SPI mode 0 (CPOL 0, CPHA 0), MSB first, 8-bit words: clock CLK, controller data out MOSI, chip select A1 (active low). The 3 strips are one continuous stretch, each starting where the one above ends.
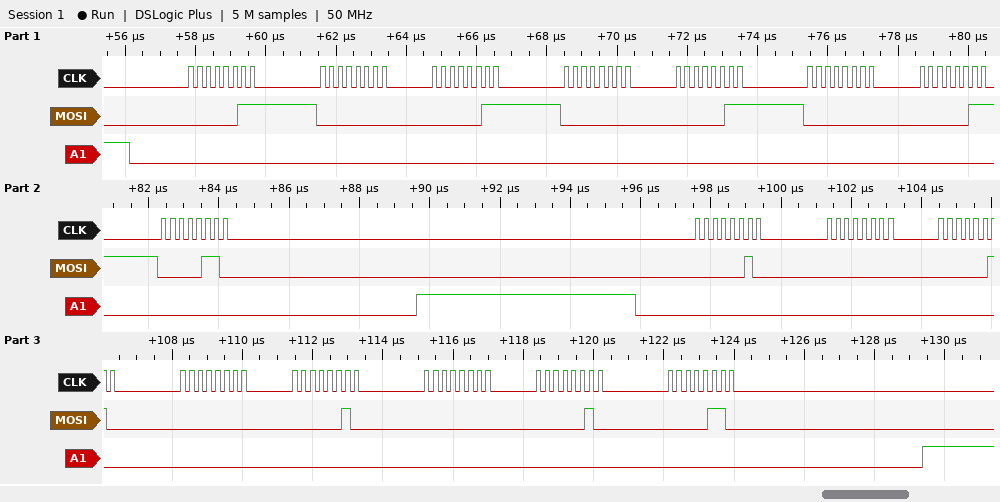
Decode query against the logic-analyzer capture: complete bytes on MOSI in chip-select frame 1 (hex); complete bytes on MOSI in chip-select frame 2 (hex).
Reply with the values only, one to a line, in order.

03 00 03 00 03 00 03 06
02 00 02 00 02 00 02 06
